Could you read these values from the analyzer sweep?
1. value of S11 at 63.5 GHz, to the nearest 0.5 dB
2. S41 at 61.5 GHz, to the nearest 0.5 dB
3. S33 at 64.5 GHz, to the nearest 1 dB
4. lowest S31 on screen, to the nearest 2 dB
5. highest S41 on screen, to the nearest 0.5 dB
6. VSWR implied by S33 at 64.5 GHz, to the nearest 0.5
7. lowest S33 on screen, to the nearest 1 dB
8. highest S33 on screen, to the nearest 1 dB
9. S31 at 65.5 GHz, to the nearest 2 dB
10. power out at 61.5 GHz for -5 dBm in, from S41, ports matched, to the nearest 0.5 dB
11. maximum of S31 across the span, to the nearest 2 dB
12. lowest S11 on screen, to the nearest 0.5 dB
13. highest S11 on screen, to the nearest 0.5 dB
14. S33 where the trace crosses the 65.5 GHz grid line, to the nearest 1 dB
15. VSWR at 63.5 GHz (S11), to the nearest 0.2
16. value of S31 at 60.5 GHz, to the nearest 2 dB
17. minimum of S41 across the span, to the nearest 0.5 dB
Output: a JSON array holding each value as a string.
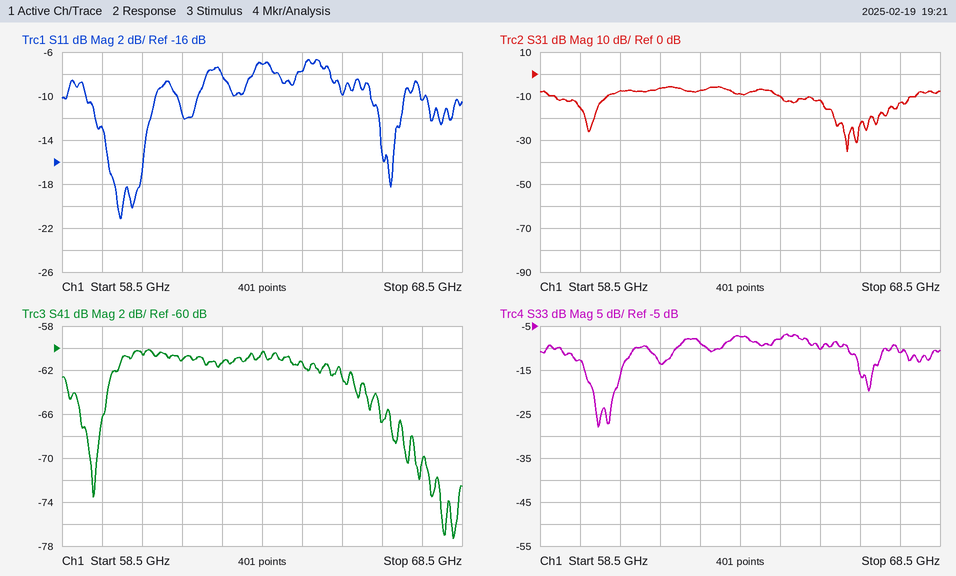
["-7.0 dB", "-61.0 dB", "-8 dB", "-36 dB", "-60.0 dB", "2.5", "-28 dB", "-7 dB", "-12 dB", "-66.0 dBm", "-6 dB", "-21.0 dB", "-6.5 dB", "-10 dB", "2.6", "-8 dB", "-77.5 dB"]
